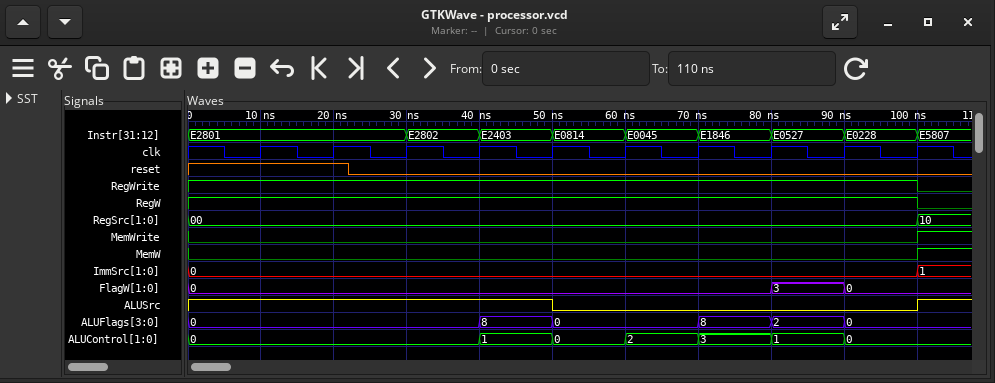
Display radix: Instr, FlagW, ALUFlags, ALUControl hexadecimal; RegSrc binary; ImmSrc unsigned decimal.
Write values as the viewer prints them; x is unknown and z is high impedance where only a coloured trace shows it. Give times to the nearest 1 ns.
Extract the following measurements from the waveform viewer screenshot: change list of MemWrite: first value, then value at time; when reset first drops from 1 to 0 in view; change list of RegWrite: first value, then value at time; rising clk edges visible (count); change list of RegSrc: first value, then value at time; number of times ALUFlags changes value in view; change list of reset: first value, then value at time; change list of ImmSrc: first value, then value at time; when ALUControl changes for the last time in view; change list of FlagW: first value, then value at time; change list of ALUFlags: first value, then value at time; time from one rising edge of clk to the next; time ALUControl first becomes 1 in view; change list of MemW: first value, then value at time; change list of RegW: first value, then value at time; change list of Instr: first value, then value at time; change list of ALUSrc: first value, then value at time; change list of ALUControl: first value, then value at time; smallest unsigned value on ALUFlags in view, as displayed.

0, 1 at 100 ns
22 ns
1, 0 at 100 ns
10
00, 10 at 100 ns
5
1, 0 at 22 ns
0, 1 at 100 ns
90 ns
0, 3 at 80 ns, 0 at 90 ns
0, 8 at 40 ns, 0 at 50 ns, 8 at 70 ns, 2 at 80 ns, 0 at 90 ns
10 ns
40 ns
0, 1 at 100 ns
1, 0 at 100 ns
E2801, E2802 at 30 ns, E2403 at 40 ns, E0814 at 50 ns, E0045 at 60 ns, E1846 at 70 ns, E0527 at 80 ns, E0228 at 90 ns, E5807 at 100 ns
1, 0 at 50 ns, 1 at 100 ns
0, 1 at 40 ns, 0 at 50 ns, 2 at 60 ns, 3 at 70 ns, 1 at 80 ns, 0 at 90 ns
0
